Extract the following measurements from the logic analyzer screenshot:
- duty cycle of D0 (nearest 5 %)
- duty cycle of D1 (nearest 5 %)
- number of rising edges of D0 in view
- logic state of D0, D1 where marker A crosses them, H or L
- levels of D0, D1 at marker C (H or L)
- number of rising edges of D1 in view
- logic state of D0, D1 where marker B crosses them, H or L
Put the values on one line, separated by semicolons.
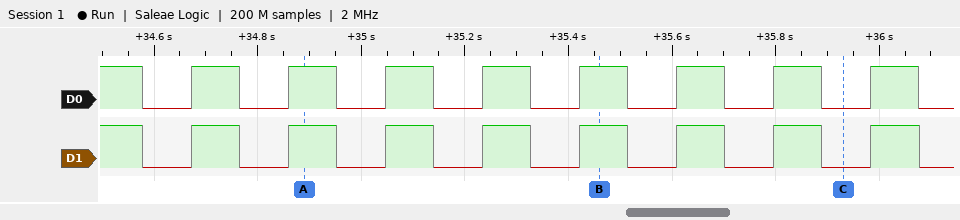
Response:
50 %; 50 %; 8; D0=H, D1=H; D0=L, D1=L; 8; D0=H, D1=H
